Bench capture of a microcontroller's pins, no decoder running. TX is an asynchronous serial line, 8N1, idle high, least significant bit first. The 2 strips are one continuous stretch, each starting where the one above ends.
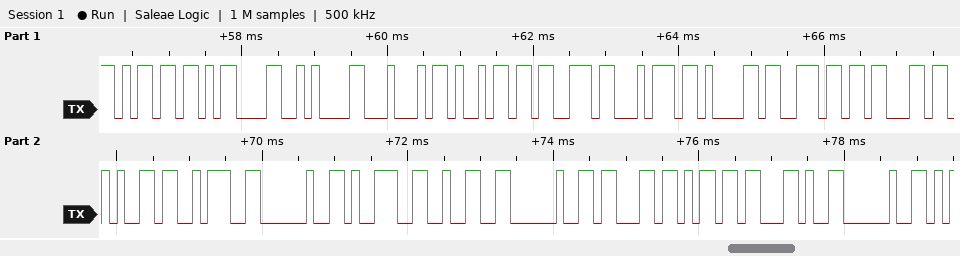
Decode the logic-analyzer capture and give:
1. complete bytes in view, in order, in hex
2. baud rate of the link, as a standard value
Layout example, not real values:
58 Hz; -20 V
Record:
6D 0D 0A 44 69 73 74 61 6E 63 65 3A 20 39 32 20 63 6D 2C 20; 9600 baud
